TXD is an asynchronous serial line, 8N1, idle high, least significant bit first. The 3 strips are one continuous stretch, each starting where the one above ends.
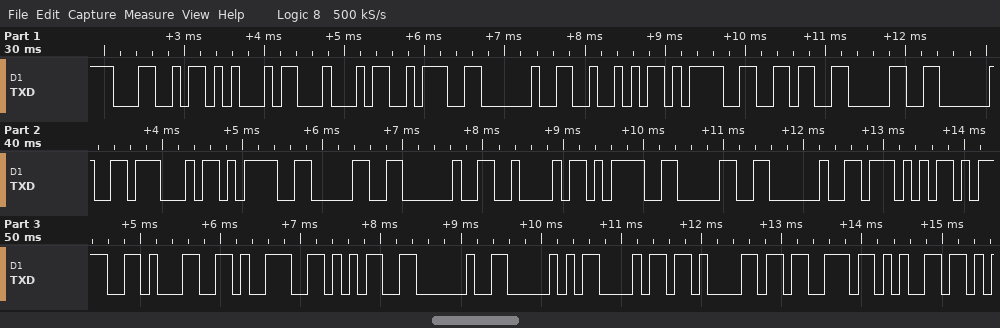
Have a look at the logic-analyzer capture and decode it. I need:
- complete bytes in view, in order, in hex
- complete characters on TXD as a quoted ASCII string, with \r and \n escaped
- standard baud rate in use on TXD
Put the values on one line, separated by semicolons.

4C 45 44 3A 20 52 3D 36 30 20 47 3D 30 20 42 3D 30 20 57 3D 31 39 35 20 50 68 61 73 65; "LED: R=60 G=0 B=0 W=195 Phase"; 9600 baud
